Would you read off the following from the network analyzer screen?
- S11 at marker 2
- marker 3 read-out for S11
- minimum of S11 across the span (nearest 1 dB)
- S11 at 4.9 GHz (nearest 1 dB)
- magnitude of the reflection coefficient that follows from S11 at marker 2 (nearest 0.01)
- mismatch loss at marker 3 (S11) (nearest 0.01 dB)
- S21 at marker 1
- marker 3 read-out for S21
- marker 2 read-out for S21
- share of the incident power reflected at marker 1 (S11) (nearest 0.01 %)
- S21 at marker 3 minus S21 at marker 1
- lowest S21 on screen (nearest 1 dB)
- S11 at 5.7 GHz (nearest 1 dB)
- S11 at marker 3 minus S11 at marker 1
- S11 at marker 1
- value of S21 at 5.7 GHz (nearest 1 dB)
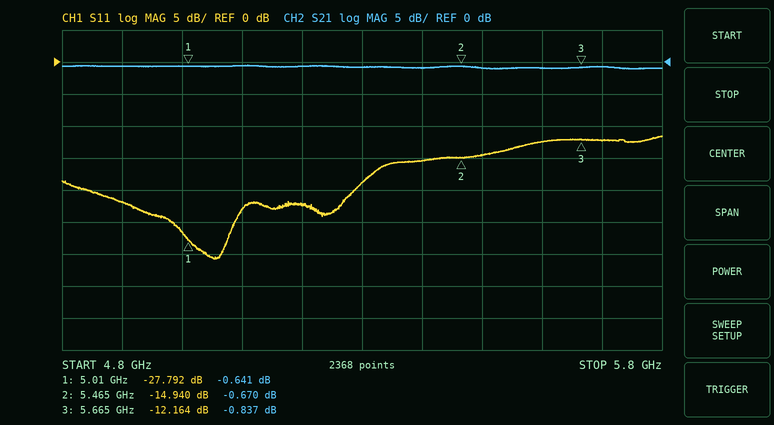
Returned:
-14.940 dB
-12.164 dB
-31 dB
-22 dB
0.18
0.27 dB
-0.641 dB
-0.837 dB
-0.670 dB
0.17 %
-0.196 dB
-1 dB
-12 dB
15.628 dB
-27.792 dB
-1 dB
